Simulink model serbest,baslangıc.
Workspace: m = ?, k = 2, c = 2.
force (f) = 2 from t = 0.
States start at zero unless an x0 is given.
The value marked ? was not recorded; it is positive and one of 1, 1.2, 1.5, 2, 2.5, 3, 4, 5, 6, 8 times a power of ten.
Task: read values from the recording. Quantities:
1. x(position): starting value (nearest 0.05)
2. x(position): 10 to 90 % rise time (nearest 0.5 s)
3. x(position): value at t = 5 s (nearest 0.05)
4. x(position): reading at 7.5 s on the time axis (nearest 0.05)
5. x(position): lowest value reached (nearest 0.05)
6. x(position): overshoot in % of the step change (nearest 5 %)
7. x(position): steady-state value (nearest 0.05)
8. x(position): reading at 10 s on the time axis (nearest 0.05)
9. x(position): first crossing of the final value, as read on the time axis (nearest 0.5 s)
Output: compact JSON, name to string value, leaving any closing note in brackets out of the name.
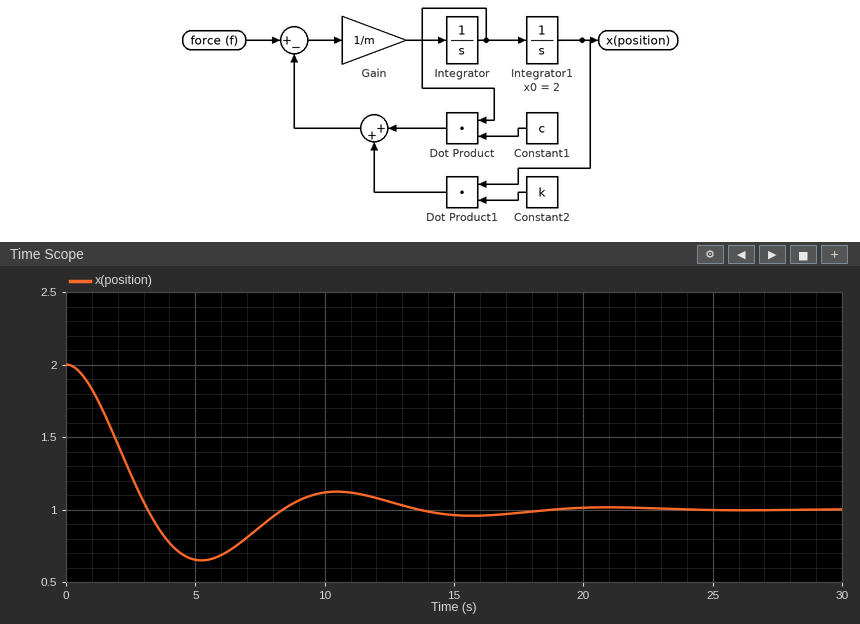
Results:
{"x(position): starting value": "2.00", "x(position): 10 to 90 % rise time": "2.0 s", "x(position): value at t = 5 s": "0.65", "x(position): reading at 7.5 s on the time axis": "0.90", "x(position): lowest value reached": "0.65", "x(position): overshoot in % of the step change": "35 %", "x(position): steady-state value": "1.00", "x(position): reading at 10 s on the time axis": "1.10", "x(position): first crossing of the final value, as read on the time axis": "3.0 s"}
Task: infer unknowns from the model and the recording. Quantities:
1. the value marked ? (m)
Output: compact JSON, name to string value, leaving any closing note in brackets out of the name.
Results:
{"the value marked ?": "5"}
